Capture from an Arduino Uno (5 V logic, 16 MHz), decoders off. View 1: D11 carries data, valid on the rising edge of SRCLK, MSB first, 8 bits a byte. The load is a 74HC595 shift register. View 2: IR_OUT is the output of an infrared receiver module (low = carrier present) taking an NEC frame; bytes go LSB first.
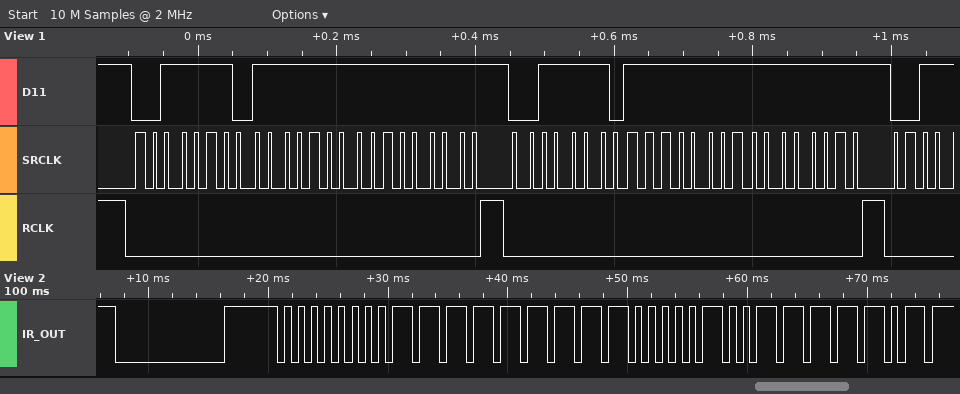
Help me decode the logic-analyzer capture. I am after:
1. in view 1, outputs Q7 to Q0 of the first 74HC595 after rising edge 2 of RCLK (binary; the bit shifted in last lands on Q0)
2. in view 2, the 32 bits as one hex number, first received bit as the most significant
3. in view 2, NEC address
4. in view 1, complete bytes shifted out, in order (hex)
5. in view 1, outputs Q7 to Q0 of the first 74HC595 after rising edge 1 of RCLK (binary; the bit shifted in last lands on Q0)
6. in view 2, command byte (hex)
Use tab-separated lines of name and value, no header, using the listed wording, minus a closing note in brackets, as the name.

in view 1, outputs Q7 to Q0 of the first 74HC595 after rising edge 2 of RCLK	11111111
in view 2, the 32 bits as one hex number, first received bit as the most significant	0x00FF827D
in view 2, NEC address	0x00
in view 1, complete bytes shifted out, in order	3E FF FF 3E FF FF
in view 1, outputs Q7 to Q0 of the first 74HC595 after rising edge 1 of RCLK	11111111
in view 2, command byte	0x41
